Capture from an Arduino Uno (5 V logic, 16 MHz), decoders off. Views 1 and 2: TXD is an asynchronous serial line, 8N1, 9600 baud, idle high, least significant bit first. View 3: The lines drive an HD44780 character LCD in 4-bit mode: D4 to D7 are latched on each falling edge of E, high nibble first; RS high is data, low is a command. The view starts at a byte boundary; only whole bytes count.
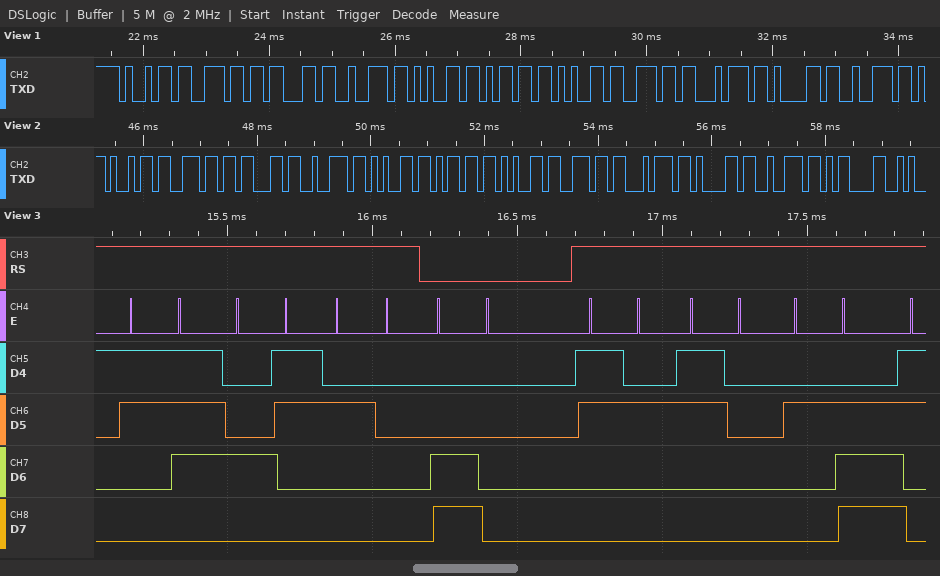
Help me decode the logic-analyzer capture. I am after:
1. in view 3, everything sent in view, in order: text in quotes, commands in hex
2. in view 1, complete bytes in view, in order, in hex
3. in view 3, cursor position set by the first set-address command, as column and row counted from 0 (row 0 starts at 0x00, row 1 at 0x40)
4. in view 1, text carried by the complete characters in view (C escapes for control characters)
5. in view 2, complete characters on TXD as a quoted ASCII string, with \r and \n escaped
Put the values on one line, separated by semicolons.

"7C " 0xC0 "20."; 69 6E 63 72 65 6D 65 6E 74 61 72; column 0, row 1; "incrementar"; "incrementar\r"
